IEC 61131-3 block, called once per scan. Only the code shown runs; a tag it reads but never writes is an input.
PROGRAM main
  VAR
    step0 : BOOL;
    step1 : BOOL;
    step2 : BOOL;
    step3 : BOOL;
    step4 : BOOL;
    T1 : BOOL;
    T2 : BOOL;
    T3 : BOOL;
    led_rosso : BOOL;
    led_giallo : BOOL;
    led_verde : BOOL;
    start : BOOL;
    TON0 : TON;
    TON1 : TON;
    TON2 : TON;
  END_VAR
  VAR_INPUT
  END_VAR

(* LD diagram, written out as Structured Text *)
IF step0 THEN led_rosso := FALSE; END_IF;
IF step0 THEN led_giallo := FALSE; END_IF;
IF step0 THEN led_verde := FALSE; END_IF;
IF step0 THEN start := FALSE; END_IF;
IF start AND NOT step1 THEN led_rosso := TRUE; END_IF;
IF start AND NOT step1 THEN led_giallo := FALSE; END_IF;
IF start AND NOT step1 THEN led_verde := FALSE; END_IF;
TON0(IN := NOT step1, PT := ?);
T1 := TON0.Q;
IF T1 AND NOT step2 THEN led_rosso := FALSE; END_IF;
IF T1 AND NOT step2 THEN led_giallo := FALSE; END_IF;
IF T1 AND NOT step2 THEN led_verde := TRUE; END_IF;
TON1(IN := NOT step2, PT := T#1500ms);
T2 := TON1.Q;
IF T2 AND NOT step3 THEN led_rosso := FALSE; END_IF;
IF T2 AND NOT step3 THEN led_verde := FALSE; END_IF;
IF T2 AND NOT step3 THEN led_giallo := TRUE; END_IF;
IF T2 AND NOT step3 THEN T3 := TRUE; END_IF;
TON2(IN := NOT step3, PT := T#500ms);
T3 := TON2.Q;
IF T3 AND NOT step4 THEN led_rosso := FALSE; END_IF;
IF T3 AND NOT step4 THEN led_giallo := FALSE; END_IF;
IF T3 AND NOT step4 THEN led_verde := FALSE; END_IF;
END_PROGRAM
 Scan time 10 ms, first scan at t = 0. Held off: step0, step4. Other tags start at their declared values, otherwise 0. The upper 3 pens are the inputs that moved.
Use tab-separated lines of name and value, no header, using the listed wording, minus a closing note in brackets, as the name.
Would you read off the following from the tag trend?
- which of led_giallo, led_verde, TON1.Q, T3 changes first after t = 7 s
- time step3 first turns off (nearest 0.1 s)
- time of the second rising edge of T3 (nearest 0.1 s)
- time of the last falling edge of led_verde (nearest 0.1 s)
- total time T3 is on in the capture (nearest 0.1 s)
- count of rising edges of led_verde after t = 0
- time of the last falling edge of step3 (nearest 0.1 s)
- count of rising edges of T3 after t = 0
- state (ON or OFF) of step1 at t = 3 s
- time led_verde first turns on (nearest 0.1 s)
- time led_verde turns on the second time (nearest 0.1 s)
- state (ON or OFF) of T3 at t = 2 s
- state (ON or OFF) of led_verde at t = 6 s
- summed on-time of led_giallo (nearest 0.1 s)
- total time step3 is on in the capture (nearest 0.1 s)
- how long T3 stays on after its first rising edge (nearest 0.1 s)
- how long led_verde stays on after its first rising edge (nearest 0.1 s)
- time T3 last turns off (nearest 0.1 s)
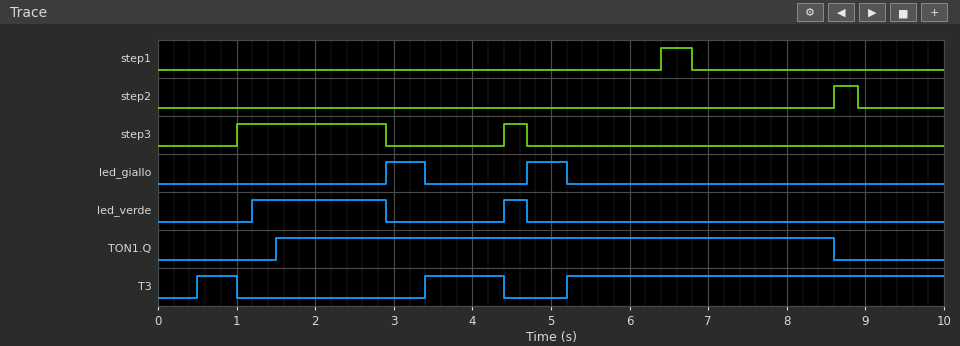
which of led_giallo, led_verde, TON1.Q, T3 changes first after t = 7 s	TON1.Q
time step3 first turns off	2.9 s
time of the second rising edge of T3	3.4 s
time of the last falling edge of led_verde	4.7 s
total time T3 is on in the capture	6.3 s
count of rising edges of led_verde after t = 0	2
time of the last falling edge of step3	4.7 s
count of rising edges of T3 after t = 0	3
state (ON or OFF) of step1 at t = 3 s	OFF
time led_verde first turns on	1.2 s
time led_verde turns on the second time	4.4 s
state (ON or OFF) of T3 at t = 2 s	OFF
state (ON or OFF) of led_verde at t = 6 s	OFF
summed on-time of led_giallo	1.0 s
total time step3 is on in the capture	2.2 s
how long T3 stays on after its first rising edge	0.5 s
how long led_verde stays on after its first rising edge	1.7 s
time T3 last turns off	4.4 s
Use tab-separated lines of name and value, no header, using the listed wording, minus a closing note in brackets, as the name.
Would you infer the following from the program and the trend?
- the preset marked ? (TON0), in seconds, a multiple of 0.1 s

the preset marked ? (TON0), in seconds, a multiple of 0.1 s	1.2 s
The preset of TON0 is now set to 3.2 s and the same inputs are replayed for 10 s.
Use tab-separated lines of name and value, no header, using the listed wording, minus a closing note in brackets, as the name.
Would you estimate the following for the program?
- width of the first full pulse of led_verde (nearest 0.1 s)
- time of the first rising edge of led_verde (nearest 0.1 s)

width of the first full pulse of led_verde	0.3 s
time of the first rising edge of led_verde	4.4 s
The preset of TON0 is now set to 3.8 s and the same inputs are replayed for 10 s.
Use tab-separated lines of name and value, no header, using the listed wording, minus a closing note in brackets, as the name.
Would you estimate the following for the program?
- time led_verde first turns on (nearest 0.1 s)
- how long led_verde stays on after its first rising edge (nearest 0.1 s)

time led_verde first turns on	4.4 s
how long led_verde stays on after its first rising edge	0.3 s
